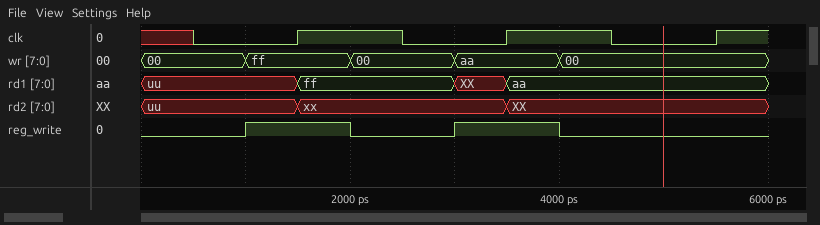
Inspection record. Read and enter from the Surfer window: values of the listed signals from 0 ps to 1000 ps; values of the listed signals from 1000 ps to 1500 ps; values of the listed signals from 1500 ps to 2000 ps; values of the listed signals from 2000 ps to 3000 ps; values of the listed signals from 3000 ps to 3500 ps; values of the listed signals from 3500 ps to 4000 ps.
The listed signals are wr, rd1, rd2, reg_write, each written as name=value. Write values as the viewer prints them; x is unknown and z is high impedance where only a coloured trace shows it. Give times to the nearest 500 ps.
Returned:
wr=00, rd1=uu, rd2=uu, reg_write=0
wr=ff, rd1=uu, rd2=uu, reg_write=1
wr=ff, rd1=ff, rd2=xx, reg_write=1
wr=00, rd1=ff, rd2=xx, reg_write=0
wr=aa, rd1=XX, rd2=xx, reg_write=1
wr=aa, rd1=aa, rd2=XX, reg_write=1
